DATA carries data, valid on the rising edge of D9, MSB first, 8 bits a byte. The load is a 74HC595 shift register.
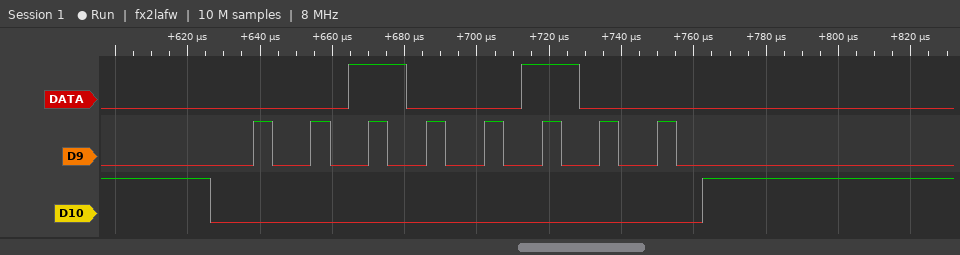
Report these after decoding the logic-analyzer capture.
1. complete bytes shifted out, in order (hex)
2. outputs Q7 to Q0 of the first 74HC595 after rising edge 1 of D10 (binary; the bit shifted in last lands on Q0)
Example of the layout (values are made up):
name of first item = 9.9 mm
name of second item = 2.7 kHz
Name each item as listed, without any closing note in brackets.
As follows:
complete bytes shifted out, in order = 24
outputs Q7 to Q0 of the first 74HC595 after rising edge 1 of D10 = 00100100
